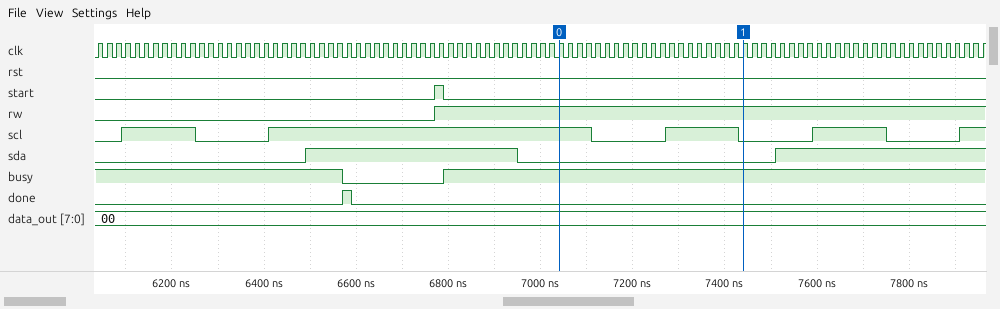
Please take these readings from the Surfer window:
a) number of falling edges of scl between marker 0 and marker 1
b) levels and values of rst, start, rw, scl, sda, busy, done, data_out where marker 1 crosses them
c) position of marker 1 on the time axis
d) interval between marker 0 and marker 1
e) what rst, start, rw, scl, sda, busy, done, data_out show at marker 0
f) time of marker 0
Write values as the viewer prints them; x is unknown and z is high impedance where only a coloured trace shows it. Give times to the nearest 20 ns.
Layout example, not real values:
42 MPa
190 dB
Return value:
2
rst=0, start=0, rw=1, scl=0, sda=0, busy=1, done=0, data_out=00
7440 ns
400 ns
rst=0, start=0, rw=1, scl=1, sda=0, busy=1, done=0, data_out=00
7040 ns
